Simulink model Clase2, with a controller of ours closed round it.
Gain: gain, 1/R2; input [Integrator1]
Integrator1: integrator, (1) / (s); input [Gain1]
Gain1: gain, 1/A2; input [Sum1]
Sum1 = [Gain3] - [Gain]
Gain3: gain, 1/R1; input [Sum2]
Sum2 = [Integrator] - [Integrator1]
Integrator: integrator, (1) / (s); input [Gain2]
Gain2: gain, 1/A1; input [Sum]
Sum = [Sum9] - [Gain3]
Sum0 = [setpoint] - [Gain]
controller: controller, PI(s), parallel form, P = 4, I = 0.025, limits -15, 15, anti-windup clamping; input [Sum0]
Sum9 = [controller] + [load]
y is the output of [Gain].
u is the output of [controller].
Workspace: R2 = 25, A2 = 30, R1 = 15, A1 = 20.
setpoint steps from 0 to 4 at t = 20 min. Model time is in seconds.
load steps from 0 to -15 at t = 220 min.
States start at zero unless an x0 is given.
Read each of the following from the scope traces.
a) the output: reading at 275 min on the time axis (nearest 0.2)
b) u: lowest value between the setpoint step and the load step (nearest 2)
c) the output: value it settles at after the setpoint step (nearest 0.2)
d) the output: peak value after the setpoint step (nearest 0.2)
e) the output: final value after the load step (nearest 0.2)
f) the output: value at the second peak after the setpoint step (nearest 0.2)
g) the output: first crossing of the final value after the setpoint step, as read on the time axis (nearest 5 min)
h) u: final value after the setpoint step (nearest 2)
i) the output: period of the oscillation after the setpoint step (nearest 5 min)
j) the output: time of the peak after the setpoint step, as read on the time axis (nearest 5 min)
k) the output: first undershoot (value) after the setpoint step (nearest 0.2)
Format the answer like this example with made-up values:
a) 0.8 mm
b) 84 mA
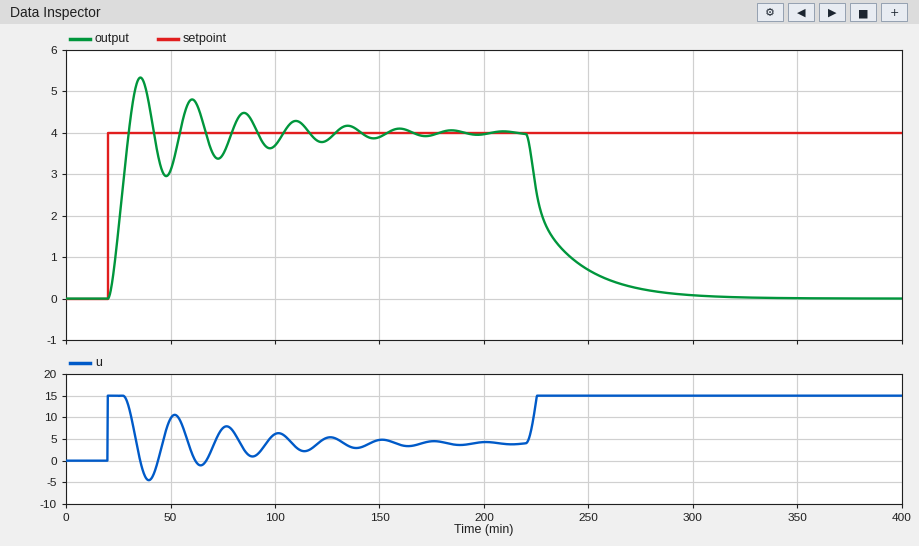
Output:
a) 0.2
b) -4
c) 4.0
d) 5.4
e) 0.0
f) 4.8
g) 30 min
h) 4
i) 25 min
j) 35 min
k) 3.0
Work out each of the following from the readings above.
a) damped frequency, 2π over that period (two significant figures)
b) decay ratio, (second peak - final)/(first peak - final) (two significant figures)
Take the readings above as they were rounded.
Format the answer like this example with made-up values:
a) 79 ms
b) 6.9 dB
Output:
a) 0.25 rad/min
b) 0.57
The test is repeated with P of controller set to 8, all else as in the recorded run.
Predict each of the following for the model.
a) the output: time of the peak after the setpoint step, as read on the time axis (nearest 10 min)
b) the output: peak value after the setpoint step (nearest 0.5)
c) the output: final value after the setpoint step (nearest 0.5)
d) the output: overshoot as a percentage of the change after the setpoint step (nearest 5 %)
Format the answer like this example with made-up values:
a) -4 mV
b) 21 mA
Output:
a) 30 min
b) 4.5
c) 4.0
d) 10 %
